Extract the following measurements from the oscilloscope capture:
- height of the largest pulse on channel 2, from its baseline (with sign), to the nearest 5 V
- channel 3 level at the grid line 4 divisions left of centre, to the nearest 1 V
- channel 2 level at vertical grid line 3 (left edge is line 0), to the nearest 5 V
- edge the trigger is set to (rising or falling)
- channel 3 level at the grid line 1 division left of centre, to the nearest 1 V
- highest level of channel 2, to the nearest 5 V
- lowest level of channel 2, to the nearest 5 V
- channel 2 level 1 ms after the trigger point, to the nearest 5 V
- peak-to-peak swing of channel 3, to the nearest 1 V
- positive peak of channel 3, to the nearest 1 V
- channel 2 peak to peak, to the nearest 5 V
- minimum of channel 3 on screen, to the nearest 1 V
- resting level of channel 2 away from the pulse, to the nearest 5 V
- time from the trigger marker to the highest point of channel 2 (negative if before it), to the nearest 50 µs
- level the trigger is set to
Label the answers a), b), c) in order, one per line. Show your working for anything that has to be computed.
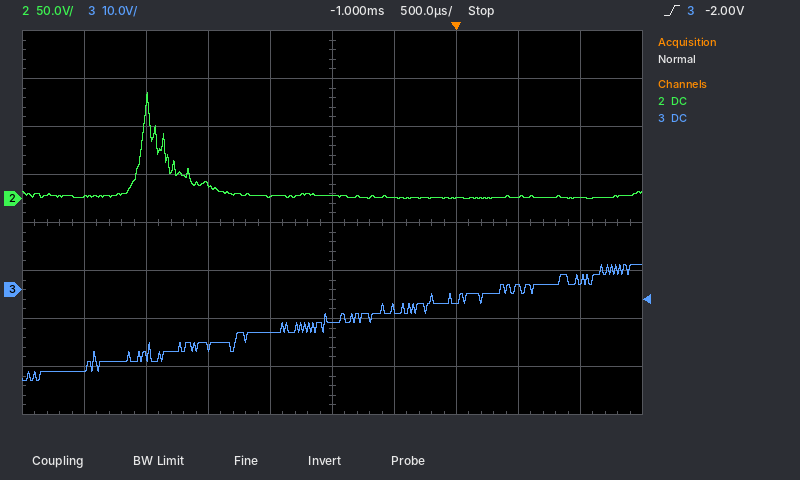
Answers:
a) 110 V − (0 V) = +110 V
b) -16 V
c) 15 V
d) rising
e) -9 V
f) 110 V
g) 0 V
h) 0 V
i) 5 V − (-19 V) = 24 V
j) 5 V
k) 110 V − (0 V) = 110 V
l) -19 V
m) 0 V
n) -2.50 ms
o) -2.00 V
